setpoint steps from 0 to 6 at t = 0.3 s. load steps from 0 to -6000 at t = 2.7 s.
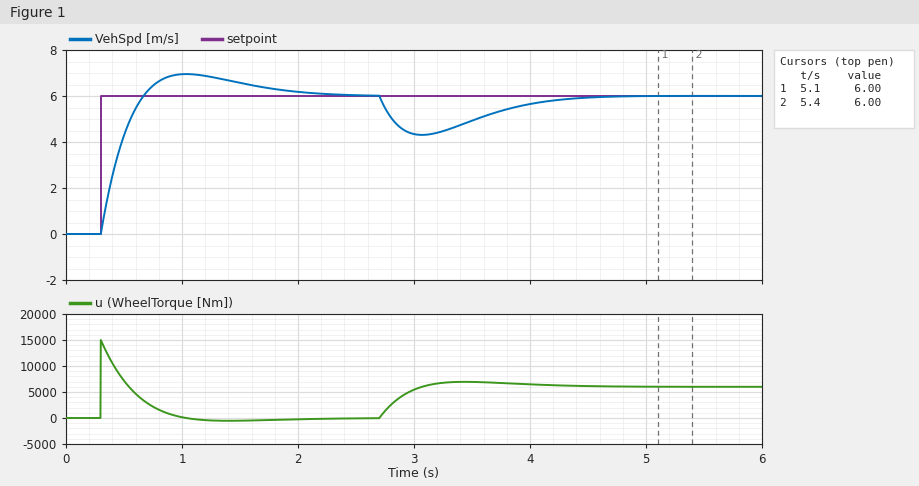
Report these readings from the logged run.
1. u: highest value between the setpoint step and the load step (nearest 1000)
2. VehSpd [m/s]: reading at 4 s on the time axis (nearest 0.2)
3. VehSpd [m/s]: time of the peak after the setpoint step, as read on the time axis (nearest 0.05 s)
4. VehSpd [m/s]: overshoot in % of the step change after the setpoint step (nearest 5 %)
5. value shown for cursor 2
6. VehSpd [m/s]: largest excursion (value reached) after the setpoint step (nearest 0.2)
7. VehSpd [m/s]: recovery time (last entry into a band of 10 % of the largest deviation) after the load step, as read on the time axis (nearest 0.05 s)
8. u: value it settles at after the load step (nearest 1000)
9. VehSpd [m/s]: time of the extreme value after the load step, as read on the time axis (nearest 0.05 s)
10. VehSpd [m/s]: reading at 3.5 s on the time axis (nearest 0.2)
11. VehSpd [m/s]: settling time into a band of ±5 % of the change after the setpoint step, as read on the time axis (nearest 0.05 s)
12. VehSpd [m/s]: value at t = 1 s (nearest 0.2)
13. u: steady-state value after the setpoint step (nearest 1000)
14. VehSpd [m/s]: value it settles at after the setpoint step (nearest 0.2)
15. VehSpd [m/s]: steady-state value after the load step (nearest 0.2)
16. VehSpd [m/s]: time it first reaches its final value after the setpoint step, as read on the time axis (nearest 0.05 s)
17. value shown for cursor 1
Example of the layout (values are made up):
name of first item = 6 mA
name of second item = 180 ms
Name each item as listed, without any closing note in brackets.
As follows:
u: highest value between the setpoint step and the load step = 15000
VehSpd [m/s]: reading at 4 s on the time axis = 5.6
VehSpd [m/s]: time of the peak after the setpoint step, as read on the time axis = 1.05 s
VehSpd [m/s]: overshoot in % of the step change after the setpoint step = 15 %
value shown for cursor 2 = 6.00
VehSpd [m/s]: largest excursion (value reached) after the setpoint step = 7.0
VehSpd [m/s]: recovery time (last entry into a band of 10 % of the largest deviation) after the load step, as read on the time axis = 4.25 s
u: value it settles at after the load step = 6000
VehSpd [m/s]: time of the extreme value after the load step, as read on the time axis = 3.05 s
VehSpd [m/s]: reading at 3.5 s on the time axis = 5.0
VehSpd [m/s]: settling time into a band of ±5 % of the change after the setpoint step, as read on the time axis = 1.80 s
VehSpd [m/s]: value at t = 1 s = 7.0
u: steady-state value after the setpoint step = 0
VehSpd [m/s]: value it settles at after the setpoint step = 6.0
VehSpd [m/s]: steady-state value after the load step = 6.0
VehSpd [m/s]: time it first reaches its final value after the setpoint step, as read on the time axis = 0.65 s
value shown for cursor 1 = 6.00
